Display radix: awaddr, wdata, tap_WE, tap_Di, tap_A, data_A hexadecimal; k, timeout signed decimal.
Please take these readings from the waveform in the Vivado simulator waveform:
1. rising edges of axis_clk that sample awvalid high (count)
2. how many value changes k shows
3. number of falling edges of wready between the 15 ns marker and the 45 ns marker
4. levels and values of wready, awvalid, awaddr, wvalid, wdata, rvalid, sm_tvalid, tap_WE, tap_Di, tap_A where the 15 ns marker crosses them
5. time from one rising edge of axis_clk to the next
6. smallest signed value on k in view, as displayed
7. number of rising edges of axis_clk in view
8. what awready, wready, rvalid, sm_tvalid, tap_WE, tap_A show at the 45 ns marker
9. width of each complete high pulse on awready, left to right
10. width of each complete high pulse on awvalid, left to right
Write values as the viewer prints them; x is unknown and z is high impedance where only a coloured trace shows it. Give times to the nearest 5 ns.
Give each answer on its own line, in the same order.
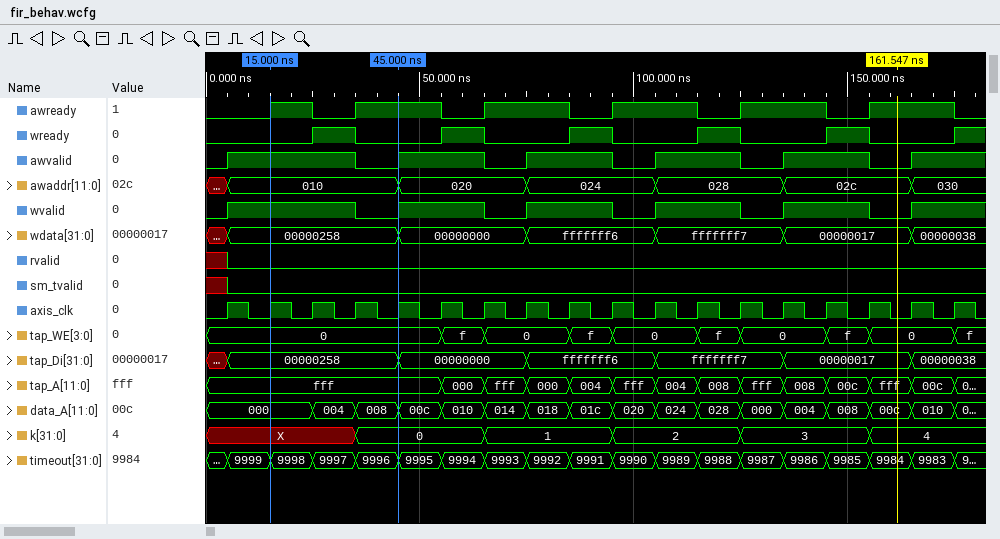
12
5
1
wready=0, awvalid=1, awaddr=010, wvalid=1, wdata=00000258, rvalid=0, sm_tvalid=0, tap_WE=0, tap_Di=00000258, tap_A=fff
10 ns
0
18
awready=1, wready=0, rvalid=0, sm_tvalid=0, tap_WE=0, tap_A=fff
10 ns, 20 ns, 20 ns, 20 ns, 20 ns, 20 ns
30 ns, 20 ns, 20 ns, 20 ns, 20 ns
